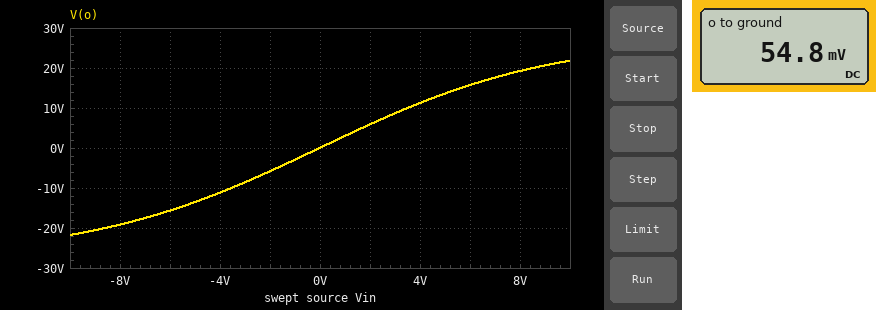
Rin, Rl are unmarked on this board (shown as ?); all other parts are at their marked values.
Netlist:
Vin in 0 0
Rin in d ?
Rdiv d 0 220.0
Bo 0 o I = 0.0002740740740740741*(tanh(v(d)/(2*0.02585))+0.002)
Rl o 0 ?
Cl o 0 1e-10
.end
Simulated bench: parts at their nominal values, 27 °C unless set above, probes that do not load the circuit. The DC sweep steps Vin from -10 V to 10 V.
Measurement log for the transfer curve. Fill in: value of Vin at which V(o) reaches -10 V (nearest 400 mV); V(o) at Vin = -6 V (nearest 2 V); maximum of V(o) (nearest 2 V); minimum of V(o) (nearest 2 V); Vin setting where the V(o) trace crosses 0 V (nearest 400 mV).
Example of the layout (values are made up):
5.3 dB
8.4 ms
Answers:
-3.6 V
-16 V
22 V
-22 V
0 V
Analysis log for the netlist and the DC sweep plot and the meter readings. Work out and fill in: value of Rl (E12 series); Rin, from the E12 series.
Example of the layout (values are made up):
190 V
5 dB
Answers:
100 kΩ
39 kΩ
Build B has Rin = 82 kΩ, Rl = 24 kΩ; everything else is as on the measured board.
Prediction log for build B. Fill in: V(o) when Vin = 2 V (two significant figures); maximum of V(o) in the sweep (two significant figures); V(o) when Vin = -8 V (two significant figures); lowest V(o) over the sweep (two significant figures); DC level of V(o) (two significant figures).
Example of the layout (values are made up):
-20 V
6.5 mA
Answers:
690 mV
3.1 V
-2.6 V
-3.1 V
13 mV
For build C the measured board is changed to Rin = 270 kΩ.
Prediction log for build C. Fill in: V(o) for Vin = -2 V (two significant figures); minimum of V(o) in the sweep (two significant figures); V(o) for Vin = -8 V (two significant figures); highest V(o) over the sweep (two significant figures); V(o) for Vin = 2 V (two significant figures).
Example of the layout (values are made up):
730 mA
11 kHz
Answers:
-810 mV
-4.2 V
-3.4 V
4.3 V
920 mV
